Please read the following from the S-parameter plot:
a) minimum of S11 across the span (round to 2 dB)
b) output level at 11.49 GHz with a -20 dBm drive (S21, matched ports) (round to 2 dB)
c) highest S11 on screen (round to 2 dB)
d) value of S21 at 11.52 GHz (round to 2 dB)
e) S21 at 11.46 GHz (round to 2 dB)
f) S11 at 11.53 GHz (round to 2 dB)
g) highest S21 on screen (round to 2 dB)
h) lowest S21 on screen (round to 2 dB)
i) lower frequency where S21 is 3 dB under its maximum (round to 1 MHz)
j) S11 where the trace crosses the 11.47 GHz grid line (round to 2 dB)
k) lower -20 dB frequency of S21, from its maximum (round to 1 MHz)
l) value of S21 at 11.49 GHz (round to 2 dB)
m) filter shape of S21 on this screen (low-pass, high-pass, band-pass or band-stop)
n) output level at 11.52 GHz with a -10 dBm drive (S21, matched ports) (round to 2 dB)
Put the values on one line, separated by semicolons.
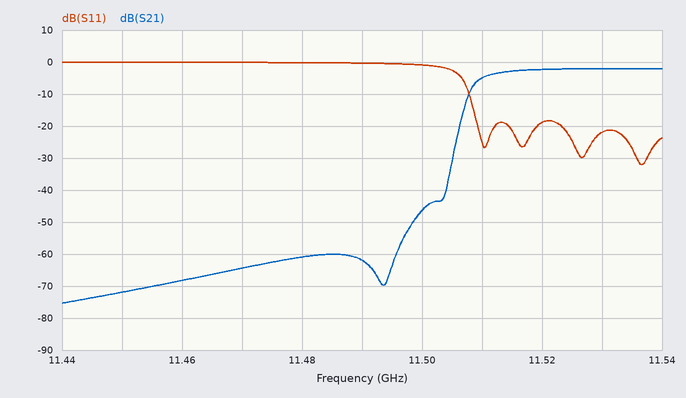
-32 dB; -82 dBm; 0 dB; -2 dB; -68 dB; -22 dB; -2 dB; -76 dB; 11.510 GHz; 0 dB; 11.506 GHz; -62 dB; high-pass; -12 dBm
